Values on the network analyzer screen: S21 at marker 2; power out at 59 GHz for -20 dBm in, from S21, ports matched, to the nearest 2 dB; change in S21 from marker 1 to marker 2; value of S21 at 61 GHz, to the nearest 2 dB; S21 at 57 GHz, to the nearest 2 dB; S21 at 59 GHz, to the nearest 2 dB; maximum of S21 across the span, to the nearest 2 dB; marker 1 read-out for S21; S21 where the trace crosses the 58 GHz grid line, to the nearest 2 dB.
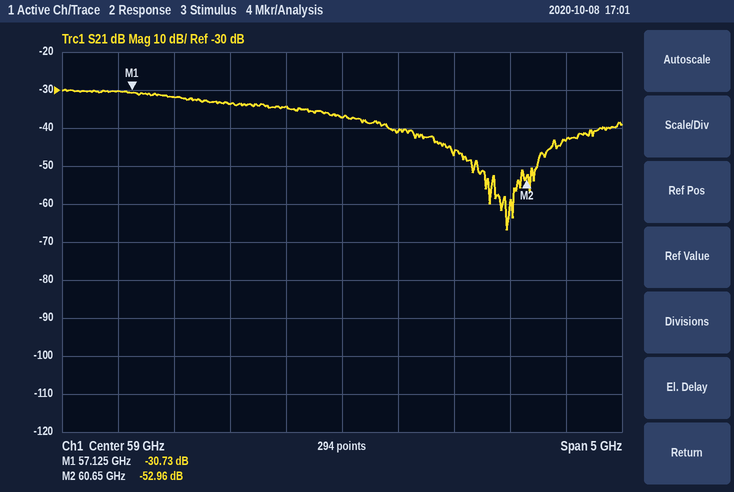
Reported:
-52.96 dB
-58 dBm
-22.23 dB
-44 dB
-30 dB
-38 dB
-30 dB
-30.73 dB
-34 dB
